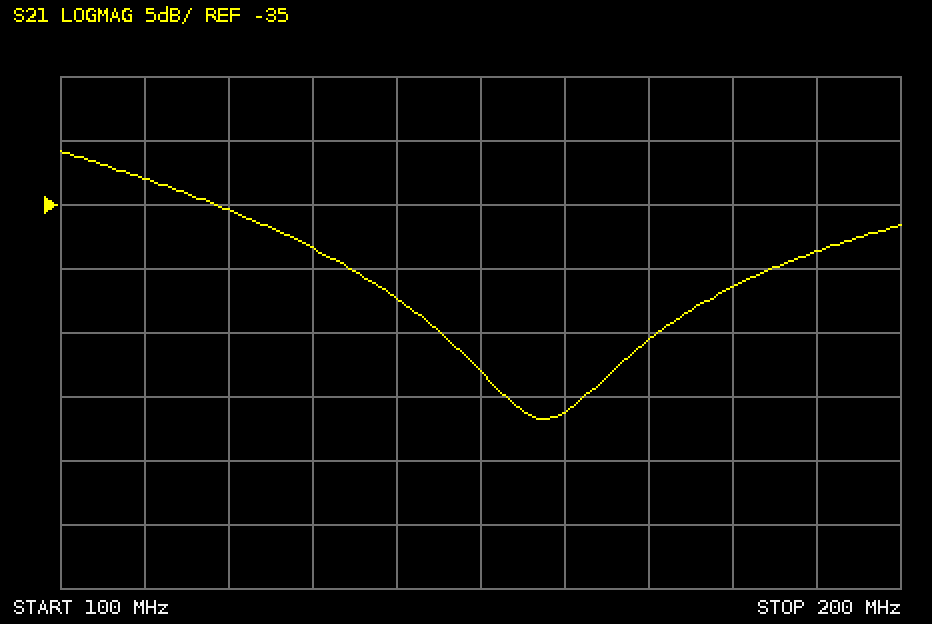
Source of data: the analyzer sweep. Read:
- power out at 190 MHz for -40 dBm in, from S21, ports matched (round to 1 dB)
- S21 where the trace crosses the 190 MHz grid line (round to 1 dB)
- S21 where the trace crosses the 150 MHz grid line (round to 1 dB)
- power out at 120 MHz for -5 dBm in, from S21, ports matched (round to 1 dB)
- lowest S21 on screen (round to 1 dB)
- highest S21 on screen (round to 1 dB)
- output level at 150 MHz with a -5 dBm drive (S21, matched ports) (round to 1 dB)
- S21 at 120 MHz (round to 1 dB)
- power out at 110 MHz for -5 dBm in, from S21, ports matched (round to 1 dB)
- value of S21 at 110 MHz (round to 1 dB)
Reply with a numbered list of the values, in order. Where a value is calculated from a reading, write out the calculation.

1. -40 dBm + (-39 dB) = -79 dBm
2. -39 dB
3. -48 dB
4. -5 dBm + (-35 dB) = -40 dBm
5. -52 dB
6. -31 dB
7. -5 dBm + (-48 dB) = -53 dBm
8. -35 dB
9. -5 dBm + (-33 dB) = -38 dBm
10. -33 dB
